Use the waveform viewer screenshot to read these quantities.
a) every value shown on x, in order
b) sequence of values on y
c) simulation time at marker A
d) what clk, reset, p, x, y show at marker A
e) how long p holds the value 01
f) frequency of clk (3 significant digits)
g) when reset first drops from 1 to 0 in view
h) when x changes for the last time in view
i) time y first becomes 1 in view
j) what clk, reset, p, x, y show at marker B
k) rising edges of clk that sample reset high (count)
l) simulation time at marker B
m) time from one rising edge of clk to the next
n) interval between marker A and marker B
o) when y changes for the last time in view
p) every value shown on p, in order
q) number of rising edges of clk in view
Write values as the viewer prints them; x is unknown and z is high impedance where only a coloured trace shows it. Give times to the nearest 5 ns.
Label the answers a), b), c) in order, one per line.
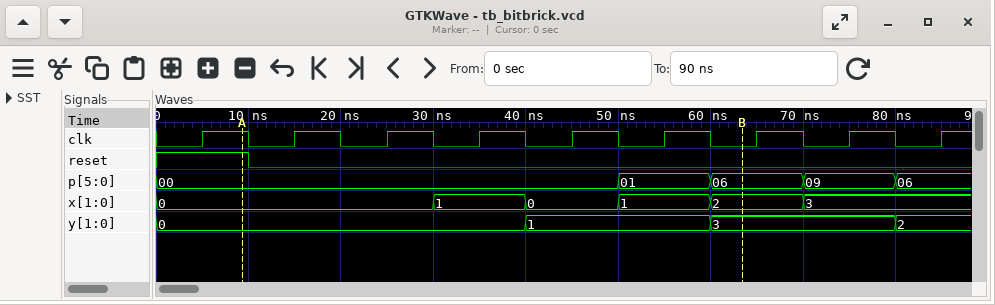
a) 0, 1, 0, 1, 2, 3
b) 0, 1, 3, 2
c) 10 ns
d) clk=1, reset=1, p=00, x=0, y=0
e) 10 ns
f) 100 MHz
g) 10 ns
h) 70 ns
i) 40 ns
j) clk=0, reset=0, p=06, x=2, y=3
k) 1
l) 65 ns
m) 10 ns
n) 55 ns
o) 80 ns
p) 00, 01, 06, 09, 06
q) 9
